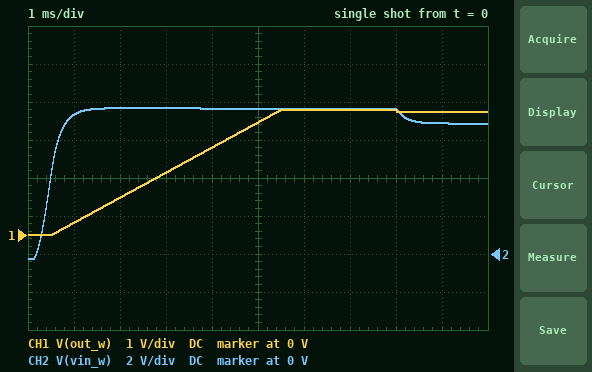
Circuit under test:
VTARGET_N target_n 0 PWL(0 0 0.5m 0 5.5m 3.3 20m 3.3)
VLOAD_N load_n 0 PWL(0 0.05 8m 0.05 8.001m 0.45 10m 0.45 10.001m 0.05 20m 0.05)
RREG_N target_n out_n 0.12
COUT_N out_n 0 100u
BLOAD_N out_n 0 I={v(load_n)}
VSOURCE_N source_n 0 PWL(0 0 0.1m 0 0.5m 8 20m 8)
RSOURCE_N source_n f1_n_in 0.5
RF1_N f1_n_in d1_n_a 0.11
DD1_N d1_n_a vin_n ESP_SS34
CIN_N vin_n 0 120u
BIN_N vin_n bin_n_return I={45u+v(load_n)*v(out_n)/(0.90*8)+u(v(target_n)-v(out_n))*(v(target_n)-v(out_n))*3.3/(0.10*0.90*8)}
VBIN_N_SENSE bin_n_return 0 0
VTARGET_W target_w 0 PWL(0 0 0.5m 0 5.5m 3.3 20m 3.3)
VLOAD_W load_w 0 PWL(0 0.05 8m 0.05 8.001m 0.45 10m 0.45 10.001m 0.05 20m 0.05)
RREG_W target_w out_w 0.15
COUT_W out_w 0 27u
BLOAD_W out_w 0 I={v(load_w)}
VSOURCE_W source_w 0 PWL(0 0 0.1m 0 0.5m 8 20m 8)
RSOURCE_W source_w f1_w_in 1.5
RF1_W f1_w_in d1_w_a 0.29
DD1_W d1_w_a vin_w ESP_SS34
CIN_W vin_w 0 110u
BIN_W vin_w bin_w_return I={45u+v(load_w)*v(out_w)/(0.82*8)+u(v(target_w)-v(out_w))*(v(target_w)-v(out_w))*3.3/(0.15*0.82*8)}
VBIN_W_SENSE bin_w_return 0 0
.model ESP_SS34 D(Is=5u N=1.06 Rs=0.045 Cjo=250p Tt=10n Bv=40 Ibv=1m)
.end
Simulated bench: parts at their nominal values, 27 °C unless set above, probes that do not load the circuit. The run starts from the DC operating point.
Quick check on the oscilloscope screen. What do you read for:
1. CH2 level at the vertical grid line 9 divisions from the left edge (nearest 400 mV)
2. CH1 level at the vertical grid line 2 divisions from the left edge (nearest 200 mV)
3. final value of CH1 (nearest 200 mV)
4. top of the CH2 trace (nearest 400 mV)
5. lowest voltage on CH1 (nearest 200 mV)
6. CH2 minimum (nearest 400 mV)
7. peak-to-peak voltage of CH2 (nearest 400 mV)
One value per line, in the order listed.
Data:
6.8 V
1.0 V
3.2 V
7.6 V
0 V
-400 mV
8.0 V
